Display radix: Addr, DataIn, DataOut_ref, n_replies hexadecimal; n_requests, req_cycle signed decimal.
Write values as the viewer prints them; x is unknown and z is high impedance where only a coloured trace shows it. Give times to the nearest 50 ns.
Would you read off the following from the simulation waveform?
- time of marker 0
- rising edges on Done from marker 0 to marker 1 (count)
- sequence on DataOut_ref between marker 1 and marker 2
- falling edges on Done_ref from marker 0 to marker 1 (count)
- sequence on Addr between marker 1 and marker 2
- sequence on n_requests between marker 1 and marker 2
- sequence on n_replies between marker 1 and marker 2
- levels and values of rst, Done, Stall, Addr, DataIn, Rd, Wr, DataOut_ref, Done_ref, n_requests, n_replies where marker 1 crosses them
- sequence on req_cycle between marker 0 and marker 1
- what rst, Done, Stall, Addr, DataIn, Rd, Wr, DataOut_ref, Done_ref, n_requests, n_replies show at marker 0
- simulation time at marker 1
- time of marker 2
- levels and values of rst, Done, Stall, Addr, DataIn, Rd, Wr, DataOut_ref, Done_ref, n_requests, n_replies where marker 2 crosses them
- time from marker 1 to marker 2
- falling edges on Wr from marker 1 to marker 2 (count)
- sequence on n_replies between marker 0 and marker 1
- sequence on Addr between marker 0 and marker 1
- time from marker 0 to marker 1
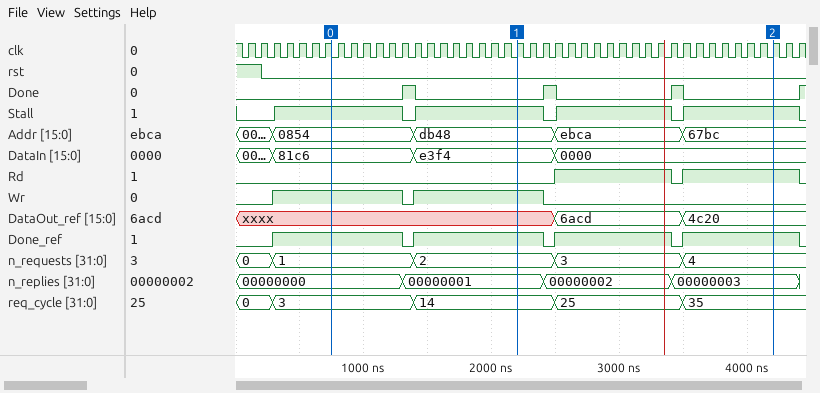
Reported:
750 ns
1
xxxx, 6acd, 4c20
1
db48, ebca, 67bc
2, 3, 4
00000001, 00000002, 00000003
rst=0, Done=0, Stall=1, Addr=db48, DataIn=e3f4, Rd=0, Wr=1, DataOut_ref=xxxx, Done_ref=1, n_requests=2, n_replies=00000001
3, 14
rst=0, Done=0, Stall=1, Addr=0854, DataIn=81c6, Rd=0, Wr=1, DataOut_ref=xxxx, Done_ref=1, n_requests=1, n_replies=00000000
2200 ns
4200 ns
rst=0, Done=0, Stall=1, Addr=67bc, DataIn=0000, Rd=1, Wr=0, DataOut_ref=4c20, Done_ref=1, n_requests=4, n_replies=00000003
2000 ns
1
00000000, 00000001
0854, db48
1450 ns
